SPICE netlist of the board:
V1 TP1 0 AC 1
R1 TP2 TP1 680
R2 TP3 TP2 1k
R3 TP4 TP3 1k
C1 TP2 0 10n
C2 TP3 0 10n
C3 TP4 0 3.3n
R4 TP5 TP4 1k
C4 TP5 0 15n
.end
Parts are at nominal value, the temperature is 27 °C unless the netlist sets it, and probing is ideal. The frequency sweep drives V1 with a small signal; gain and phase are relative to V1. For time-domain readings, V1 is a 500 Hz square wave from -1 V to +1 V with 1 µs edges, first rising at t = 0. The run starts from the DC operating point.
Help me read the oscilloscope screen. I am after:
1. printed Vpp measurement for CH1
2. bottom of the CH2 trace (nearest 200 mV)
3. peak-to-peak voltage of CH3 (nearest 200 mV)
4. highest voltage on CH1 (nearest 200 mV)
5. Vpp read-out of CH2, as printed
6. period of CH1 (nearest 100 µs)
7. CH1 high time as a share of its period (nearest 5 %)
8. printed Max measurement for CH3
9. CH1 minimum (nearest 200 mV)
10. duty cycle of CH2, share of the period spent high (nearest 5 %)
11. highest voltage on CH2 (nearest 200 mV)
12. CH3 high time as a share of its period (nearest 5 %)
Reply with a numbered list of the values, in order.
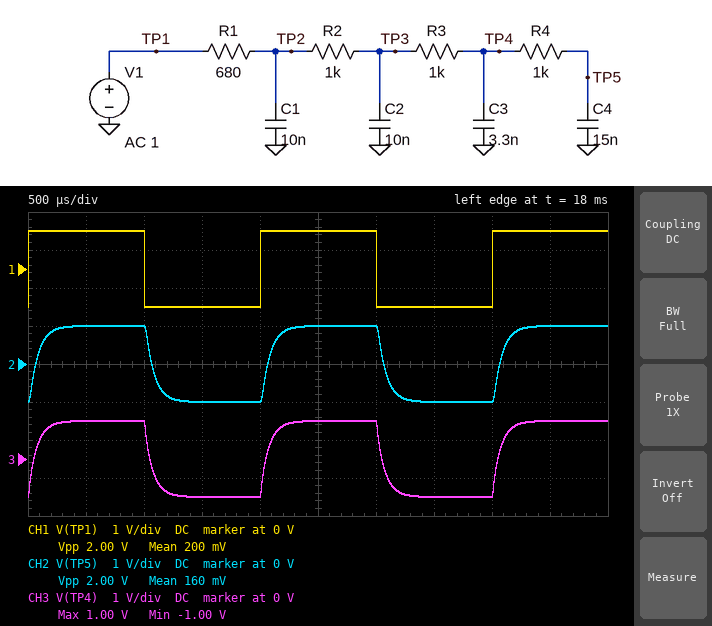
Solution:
1. 2.00 V
2. -1.0 V
3. 2.0 V
4. 1.0 V
5. 2.00 V
6. 2.0 ms
7. 50 %
8. 1.00 V
9. -1.0 V
10. 50 %
11. 1.0 V
12. 50 %
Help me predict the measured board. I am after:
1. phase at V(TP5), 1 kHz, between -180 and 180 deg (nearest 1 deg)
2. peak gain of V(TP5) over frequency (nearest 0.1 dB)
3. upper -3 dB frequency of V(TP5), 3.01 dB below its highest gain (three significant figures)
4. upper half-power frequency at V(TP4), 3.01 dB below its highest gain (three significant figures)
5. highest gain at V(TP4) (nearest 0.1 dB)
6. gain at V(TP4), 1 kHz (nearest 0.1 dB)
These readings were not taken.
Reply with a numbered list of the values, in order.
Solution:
1. -30 deg
2. 0 dB
3. 2.13 kHz
4. 2.22 kHz
5. 0 dB
6. -0.8 dB
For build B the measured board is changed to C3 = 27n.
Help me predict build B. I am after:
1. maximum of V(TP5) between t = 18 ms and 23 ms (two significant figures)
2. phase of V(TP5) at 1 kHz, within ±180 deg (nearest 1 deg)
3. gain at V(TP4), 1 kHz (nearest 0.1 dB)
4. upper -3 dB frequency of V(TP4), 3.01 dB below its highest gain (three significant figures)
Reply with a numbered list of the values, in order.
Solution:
1. 1.0 V
2. -47 deg
3. -2.2 dB
4. 1.22 kHz
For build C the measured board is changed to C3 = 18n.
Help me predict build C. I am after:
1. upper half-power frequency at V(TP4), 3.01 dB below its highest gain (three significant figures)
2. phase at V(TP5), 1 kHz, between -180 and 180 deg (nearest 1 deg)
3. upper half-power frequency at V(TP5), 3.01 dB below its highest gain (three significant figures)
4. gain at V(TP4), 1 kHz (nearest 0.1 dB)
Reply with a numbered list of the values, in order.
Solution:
1. 1.48 kHz
2. -41 deg
3. 1.45 kHz
4. -1.6 dB
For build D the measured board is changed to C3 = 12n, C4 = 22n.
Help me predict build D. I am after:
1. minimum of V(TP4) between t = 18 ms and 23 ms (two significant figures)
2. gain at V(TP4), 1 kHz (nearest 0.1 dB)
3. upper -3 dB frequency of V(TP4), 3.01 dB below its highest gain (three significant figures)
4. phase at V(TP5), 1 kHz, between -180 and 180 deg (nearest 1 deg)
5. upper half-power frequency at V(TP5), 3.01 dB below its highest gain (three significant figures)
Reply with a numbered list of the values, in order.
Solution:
1. -1.0 V
2. -1.8 dB
3. 1.38 kHz
4. -43 deg
5. 1.34 kHz
